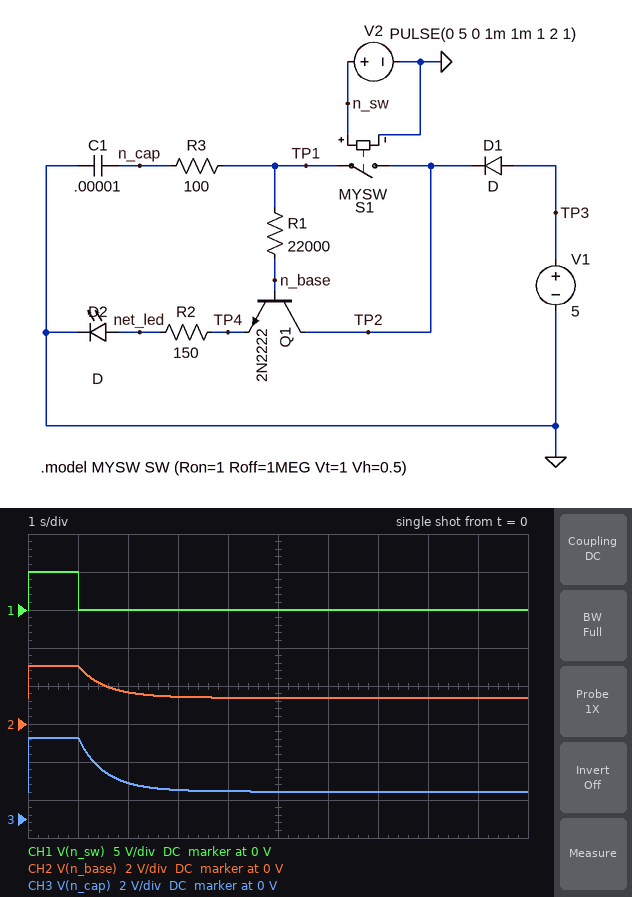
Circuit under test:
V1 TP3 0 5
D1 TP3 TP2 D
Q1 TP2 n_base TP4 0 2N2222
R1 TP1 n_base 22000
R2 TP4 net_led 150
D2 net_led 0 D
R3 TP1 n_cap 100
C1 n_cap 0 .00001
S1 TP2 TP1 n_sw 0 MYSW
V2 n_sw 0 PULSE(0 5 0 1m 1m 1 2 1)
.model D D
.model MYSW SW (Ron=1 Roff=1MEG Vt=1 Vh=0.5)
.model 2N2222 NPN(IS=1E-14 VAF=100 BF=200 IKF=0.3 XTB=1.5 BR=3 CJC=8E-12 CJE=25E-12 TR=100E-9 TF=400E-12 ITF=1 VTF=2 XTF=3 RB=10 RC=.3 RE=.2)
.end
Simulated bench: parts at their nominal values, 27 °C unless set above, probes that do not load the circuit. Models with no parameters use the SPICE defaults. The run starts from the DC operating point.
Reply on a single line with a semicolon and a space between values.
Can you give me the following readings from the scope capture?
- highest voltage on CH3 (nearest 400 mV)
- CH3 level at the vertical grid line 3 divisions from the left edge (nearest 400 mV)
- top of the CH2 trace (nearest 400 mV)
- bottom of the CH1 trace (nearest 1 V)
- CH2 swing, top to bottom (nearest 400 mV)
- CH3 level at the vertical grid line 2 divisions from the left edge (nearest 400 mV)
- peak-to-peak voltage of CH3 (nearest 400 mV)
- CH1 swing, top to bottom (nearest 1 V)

4.4 V; 1.6 V; 3.2 V; 0 V; 1.6 V; 2.0 V; 2.8 V; 5 V
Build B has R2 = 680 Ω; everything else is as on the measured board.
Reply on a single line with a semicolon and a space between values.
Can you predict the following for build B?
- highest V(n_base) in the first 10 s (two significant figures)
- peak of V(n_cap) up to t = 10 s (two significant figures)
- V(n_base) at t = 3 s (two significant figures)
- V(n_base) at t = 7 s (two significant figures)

3.9 V; 4.3 V; 2.2 V; 1.7 V
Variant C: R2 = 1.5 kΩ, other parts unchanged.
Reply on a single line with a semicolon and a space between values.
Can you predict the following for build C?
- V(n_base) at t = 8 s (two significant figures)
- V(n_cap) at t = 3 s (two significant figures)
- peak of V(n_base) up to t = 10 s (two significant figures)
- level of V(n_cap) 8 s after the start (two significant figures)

2.1 V; 3.1 V; 4.1 V; 2.2 V
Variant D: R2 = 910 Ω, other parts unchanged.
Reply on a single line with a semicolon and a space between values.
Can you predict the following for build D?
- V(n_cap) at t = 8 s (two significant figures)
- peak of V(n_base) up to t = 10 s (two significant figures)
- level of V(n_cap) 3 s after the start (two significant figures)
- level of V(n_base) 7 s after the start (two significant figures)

1.9 V; 4.0 V; 2.6 V; 1.8 V
